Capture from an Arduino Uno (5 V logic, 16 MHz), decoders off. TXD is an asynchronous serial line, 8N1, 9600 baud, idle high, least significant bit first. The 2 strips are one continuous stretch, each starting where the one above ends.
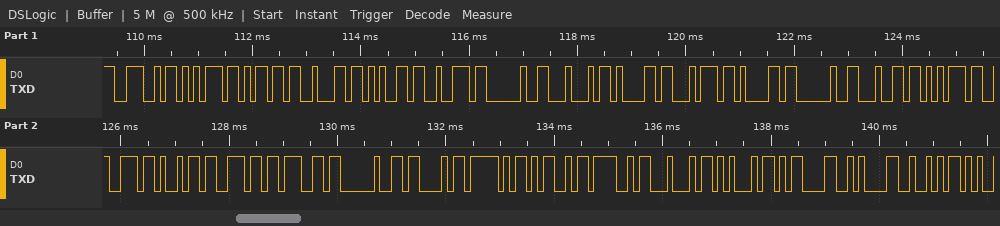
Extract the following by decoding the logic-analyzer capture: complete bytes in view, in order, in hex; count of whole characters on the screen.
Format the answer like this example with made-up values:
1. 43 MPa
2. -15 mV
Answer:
1. 4E 75 6D 62 65 72 20 44 61 74 61 20 64 75 72 69 6E 67 20 43 5F 4D 4F 44 45 0D 0A 52
2. 28
